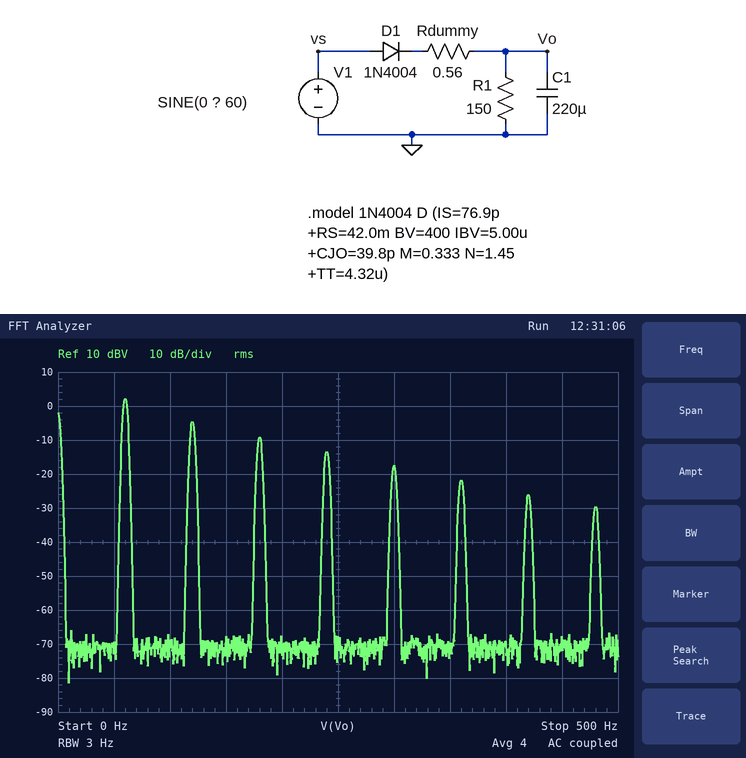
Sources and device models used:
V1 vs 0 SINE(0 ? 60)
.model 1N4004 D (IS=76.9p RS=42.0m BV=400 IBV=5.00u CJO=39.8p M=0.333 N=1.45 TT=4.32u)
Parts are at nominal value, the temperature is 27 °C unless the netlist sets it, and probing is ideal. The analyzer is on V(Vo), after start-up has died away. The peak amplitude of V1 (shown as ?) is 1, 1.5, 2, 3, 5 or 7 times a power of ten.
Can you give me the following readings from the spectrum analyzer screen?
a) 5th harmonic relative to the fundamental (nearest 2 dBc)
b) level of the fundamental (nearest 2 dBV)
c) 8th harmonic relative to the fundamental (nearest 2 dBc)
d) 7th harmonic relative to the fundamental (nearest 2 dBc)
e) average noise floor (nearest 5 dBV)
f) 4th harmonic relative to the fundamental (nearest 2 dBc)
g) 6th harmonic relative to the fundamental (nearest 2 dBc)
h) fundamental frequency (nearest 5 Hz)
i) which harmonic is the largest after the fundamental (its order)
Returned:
-20 dBc
2 dBV
-32 dBc
-28 dBc
-70 dBV
-16 dBc
-24 dBc
60 Hz
2
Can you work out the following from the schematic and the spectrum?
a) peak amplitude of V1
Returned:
15 V
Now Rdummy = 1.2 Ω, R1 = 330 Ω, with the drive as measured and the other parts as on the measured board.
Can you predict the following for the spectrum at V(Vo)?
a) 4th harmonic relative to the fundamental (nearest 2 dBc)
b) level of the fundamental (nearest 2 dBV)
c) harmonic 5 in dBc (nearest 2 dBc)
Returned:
-14 dBc
-4 dBV
-18 dBc
